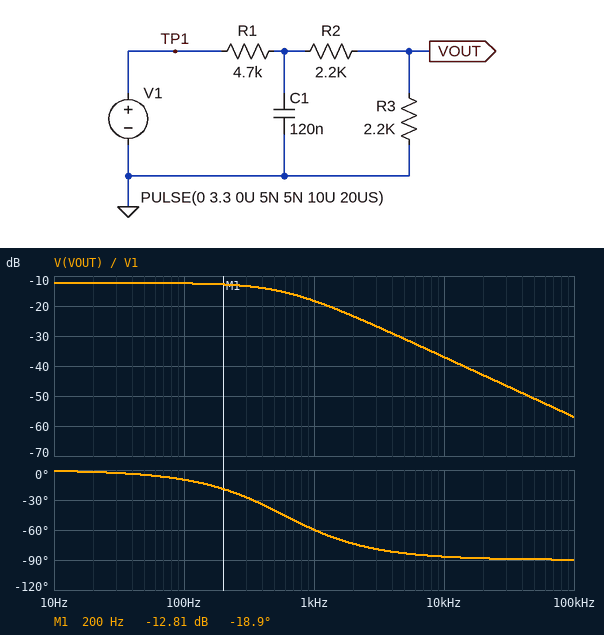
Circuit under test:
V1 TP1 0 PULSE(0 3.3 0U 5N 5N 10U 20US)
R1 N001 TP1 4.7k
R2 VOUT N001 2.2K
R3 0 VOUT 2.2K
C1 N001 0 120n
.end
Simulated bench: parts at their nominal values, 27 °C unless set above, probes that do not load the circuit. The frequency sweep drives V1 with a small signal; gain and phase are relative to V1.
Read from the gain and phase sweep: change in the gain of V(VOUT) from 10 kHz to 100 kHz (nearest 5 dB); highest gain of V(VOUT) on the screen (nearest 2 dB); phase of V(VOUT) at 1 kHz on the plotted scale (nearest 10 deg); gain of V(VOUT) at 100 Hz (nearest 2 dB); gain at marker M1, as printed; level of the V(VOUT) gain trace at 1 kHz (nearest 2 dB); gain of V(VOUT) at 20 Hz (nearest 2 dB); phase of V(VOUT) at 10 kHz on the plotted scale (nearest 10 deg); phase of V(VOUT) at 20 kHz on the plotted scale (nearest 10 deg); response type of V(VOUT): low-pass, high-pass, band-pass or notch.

-20 dB
-12 dB
-60 deg
-12 dB
-12.81 dB
-18 dB
-12 dB
-90 deg
-90 deg
low-pass
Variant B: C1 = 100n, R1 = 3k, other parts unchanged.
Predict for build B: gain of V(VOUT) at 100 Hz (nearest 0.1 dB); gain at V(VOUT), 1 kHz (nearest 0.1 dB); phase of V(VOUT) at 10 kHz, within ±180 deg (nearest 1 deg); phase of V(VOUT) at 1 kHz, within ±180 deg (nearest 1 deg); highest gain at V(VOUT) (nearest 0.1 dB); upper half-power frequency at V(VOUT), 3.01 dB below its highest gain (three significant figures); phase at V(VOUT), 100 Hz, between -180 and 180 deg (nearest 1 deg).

-10.6 dB
-14.1 dB
-85 deg
-48 deg
-10.5 dB
892 Hz
-6 deg
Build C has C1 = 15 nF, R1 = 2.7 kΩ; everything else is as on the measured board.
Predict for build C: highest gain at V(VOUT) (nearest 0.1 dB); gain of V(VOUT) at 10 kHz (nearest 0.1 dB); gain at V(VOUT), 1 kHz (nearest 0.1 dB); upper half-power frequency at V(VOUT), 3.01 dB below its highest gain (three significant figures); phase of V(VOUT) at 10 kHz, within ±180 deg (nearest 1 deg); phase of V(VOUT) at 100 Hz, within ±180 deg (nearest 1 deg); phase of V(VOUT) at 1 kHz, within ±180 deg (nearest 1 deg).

-10.2 dB
-15.6 dB
-10.3 dB
6.34 kHz
-58 deg
-1 deg
-9 deg
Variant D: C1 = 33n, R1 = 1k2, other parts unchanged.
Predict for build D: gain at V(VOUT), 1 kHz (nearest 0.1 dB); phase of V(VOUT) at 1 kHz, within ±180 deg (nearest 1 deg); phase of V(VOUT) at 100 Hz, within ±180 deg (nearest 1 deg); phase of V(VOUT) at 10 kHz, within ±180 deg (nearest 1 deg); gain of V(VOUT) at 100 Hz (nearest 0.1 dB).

-8.3 dB
-11 deg
-1 deg
-63 deg
-8.1 dB
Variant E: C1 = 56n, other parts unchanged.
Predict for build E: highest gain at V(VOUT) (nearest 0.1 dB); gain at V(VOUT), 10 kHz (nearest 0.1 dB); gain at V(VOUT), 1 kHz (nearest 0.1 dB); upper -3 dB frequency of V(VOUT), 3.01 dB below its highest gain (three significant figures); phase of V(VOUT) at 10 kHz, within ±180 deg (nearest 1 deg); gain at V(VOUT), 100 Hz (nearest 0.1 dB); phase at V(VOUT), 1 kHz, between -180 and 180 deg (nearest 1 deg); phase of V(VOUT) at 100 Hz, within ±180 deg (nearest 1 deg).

-12.3 dB
-30.5 dB
-14.5 dB
1.25 kHz
-83 deg
-12.4 dB
-39 deg
-5 deg
